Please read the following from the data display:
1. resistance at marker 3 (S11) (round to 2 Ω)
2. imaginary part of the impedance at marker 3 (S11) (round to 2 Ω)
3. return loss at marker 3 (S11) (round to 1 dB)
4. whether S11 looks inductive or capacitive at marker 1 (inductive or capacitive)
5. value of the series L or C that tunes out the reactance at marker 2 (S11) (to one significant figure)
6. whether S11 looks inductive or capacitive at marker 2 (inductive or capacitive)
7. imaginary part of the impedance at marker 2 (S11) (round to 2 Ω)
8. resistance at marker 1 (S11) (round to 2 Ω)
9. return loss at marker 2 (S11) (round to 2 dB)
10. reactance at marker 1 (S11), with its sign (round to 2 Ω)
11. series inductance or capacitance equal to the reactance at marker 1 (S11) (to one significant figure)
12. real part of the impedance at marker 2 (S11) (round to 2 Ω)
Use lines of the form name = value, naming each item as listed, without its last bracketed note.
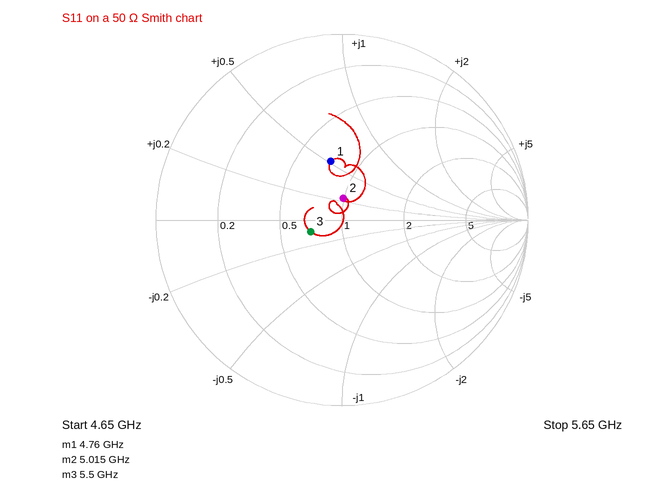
resistance at marker 3 (S11) = 36 Ω
imaginary part of the impedance at marker 3 (S11) = -4 Ω
return loss at marker 3 (S11) = 15 dB
whether S11 looks inductive or capacitive at marker 1 = inductive
value of the series L or C that tunes out the reactance at marker 2 (S11) = 3 pF
whether S11 looks inductive or capacitive at marker 2 = inductive
imaginary part of the impedance at marker 2 (S11) = +12 Ω
resistance at marker 1 (S11) = 36 Ω
return loss at marker 2 (S11) = 18 dB
reactance at marker 1 (S11), with its sign = +26 Ω
series inductance or capacitance equal to the reactance at marker 1 (S11) = 900 pH
real part of the impedance at marker 2 (S11) = 50 Ω
